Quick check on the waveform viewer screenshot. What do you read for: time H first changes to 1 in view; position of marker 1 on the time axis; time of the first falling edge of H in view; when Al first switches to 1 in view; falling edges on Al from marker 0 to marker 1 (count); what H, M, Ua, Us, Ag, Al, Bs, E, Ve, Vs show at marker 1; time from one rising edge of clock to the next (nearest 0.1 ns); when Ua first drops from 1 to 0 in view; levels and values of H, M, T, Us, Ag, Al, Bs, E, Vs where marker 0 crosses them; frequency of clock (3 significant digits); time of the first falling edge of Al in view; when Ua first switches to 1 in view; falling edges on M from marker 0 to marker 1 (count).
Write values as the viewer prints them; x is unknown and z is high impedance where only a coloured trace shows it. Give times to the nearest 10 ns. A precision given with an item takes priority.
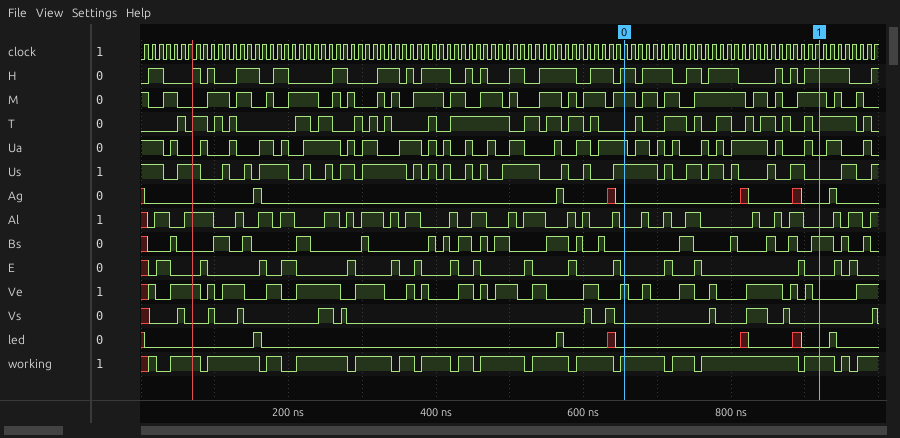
10 ns
920 ns
30 ns
20 ns
6
H=1, M=1, Ua=0, Us=0, Ag=0, Al=0, Bs=1, E=0, Ve=0, Vs=0
10 ns
30 ns
H=1, M=1, T=0, Us=1, Ag=0, Al=0, Bs=0, E=0, Vs=0
100 MHz
40 ns
40 ns
6
